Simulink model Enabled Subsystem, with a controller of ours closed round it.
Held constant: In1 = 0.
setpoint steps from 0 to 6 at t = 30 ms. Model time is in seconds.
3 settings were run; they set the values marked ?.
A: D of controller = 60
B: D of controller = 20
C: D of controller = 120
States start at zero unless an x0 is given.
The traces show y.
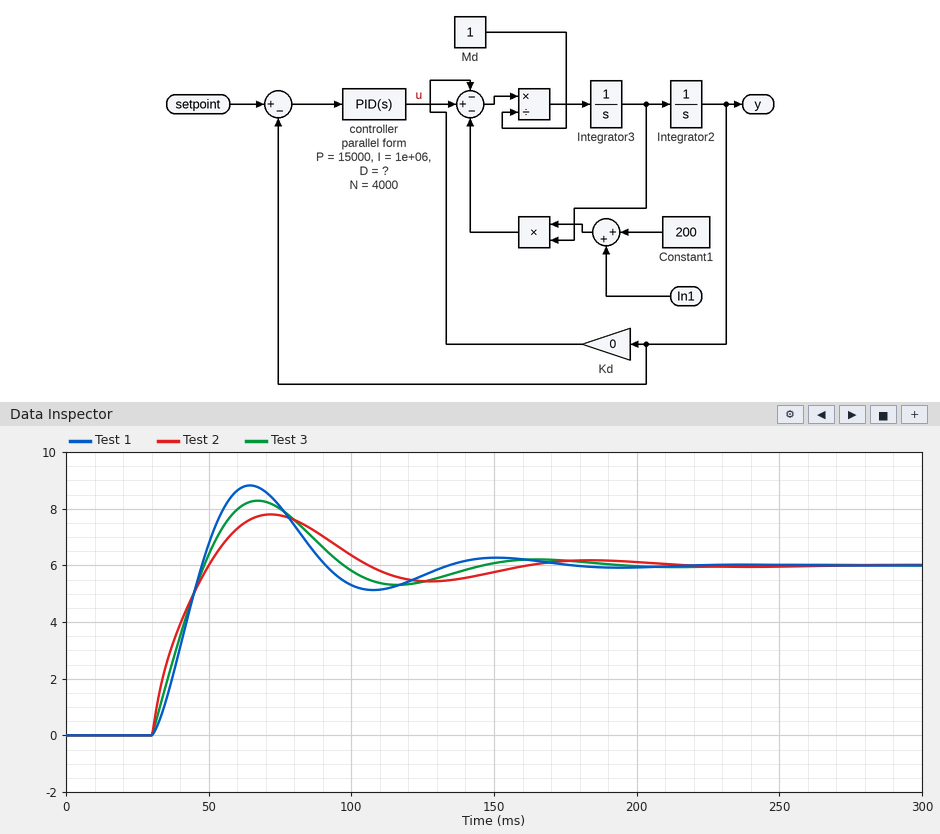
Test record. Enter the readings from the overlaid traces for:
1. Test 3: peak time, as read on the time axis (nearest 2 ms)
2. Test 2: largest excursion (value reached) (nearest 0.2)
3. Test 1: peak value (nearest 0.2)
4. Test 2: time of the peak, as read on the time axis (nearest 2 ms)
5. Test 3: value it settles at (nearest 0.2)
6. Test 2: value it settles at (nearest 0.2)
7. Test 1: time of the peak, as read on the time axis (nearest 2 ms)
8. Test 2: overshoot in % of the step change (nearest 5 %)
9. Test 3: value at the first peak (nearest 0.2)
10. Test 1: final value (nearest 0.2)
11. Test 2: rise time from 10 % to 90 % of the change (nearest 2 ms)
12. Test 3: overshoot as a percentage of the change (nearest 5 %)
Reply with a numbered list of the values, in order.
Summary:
1. 68 ms
2. 7.8
3. 8.8
4. 72 ms
5. 6.0
6. 6.0
7. 64 ms
8. 30 %
9. 8.2
10. 6.0
11. 16 ms
12. 40 %
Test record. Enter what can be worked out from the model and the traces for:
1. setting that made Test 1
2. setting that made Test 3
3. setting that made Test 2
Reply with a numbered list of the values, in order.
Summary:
1. B
2. A
3. C
